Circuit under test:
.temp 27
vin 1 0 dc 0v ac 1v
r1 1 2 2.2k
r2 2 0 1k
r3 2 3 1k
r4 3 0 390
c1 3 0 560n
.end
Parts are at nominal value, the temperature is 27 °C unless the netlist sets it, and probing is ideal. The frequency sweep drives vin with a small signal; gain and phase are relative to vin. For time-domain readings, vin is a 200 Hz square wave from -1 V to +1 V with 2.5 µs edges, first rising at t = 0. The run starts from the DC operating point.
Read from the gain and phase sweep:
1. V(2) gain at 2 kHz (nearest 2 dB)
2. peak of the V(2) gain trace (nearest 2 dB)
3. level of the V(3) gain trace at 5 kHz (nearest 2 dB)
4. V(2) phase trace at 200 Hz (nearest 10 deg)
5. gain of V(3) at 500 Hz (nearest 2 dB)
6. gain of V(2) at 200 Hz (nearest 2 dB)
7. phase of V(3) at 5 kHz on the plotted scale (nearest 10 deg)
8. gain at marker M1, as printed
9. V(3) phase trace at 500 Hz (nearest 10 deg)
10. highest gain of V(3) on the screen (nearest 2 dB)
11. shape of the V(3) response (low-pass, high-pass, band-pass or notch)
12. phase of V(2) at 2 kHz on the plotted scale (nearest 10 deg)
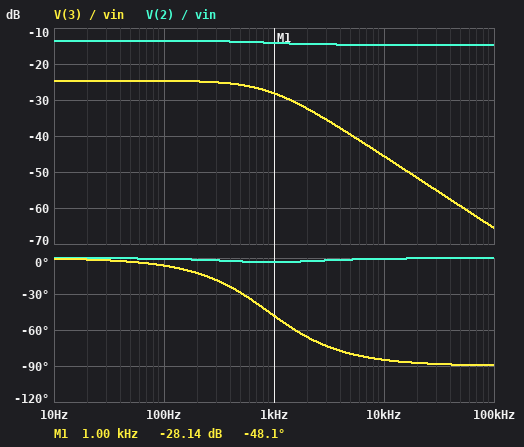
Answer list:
-14 dB
-14 dB
-40 dB
0 deg
-26 dB
-14 dB
-80 deg
-28.14 dB
-30 deg
-24 dB
low-pass
0 deg
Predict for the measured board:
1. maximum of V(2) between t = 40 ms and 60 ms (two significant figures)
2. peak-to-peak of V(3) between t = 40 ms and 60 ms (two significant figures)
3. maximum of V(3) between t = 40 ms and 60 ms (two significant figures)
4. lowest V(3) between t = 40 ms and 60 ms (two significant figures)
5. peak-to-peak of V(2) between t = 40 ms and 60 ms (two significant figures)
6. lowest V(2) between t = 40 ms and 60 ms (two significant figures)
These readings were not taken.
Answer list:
210 mV
120 mV
59 mV
-59 mV
420 mV
-210 mV
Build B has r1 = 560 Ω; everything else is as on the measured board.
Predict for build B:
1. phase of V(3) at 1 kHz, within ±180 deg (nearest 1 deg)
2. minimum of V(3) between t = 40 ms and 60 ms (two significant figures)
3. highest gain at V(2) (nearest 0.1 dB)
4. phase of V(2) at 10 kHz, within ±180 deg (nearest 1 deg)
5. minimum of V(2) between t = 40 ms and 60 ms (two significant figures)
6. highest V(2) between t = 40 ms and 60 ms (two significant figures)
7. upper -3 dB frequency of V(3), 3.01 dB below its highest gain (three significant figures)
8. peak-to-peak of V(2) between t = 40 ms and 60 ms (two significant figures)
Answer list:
-47 deg
-140 mV
-5.9 dB
0 deg
-510 mV
510 mV
938 Hz
1.0 V
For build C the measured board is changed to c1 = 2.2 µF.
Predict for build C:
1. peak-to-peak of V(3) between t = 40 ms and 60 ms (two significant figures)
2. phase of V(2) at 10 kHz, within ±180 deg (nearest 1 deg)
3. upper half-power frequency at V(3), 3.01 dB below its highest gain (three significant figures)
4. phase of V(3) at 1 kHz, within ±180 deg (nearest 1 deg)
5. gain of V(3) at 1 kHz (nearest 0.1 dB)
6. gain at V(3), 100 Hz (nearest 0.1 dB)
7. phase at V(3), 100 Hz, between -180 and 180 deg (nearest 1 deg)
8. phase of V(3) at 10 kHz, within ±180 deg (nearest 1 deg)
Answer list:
110 mV
0 deg
228 Hz
-77 deg
-37.7 dB
-25.4 dB
-24 deg
-89 deg
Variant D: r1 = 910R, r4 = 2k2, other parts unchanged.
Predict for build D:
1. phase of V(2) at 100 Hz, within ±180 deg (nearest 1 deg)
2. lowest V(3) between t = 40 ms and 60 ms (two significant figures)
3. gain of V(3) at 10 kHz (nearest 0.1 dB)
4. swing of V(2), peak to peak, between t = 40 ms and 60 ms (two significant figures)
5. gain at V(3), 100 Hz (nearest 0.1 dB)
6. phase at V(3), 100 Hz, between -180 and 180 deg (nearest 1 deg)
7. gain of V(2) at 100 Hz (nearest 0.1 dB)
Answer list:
-4 deg
-310 mV
-39.9 dB
910 mV
-10.5 dB
-17 deg
-7.0 dB
